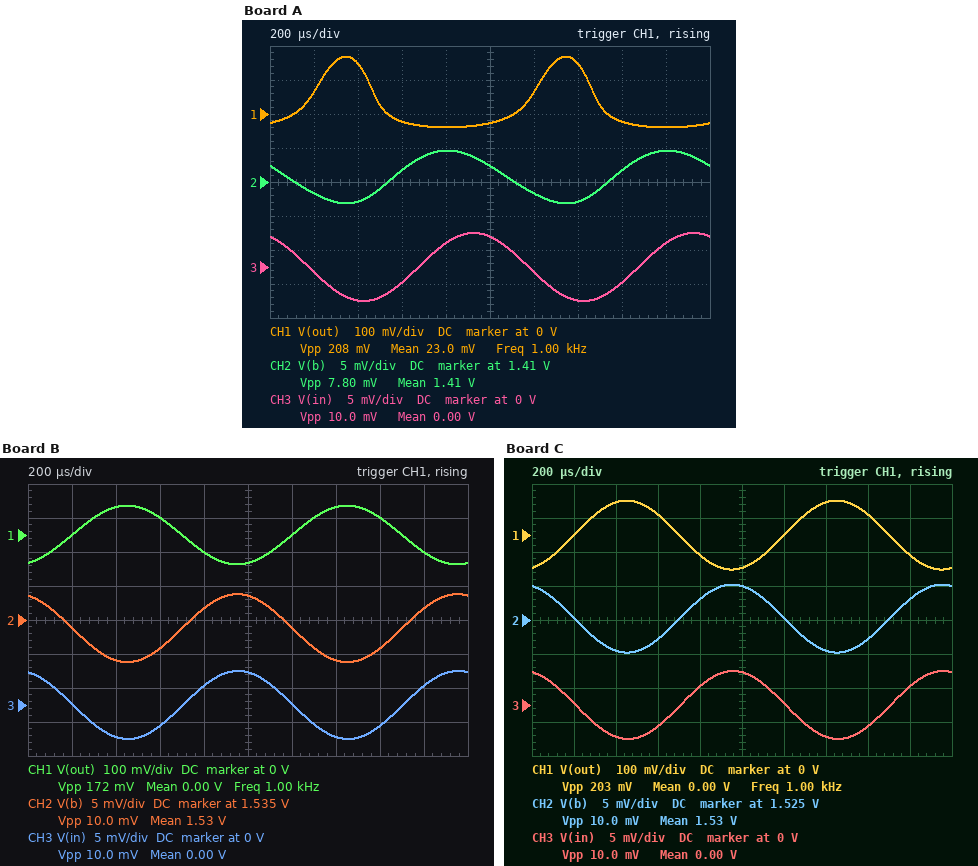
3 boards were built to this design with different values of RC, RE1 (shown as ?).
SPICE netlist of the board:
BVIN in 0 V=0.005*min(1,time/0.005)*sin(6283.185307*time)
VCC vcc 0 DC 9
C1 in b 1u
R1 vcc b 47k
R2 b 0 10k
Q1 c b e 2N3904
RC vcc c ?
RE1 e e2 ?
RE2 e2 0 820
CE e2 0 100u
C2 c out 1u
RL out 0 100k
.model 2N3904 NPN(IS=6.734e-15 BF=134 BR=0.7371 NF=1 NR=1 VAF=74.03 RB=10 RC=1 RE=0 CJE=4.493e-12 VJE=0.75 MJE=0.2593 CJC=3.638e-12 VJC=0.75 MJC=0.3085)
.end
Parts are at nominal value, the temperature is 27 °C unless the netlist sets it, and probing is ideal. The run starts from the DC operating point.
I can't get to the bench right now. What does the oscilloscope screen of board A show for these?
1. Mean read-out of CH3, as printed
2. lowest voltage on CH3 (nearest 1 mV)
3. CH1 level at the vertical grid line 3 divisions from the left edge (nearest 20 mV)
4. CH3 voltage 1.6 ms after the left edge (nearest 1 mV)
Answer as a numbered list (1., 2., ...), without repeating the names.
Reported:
1. 0.00 V
2. -5 mV
3. -20 mV
4. -2 mV
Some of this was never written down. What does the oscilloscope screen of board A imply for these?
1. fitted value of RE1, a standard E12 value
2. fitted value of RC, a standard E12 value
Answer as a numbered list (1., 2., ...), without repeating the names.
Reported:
1. 82 Ω
2. 10 kΩ
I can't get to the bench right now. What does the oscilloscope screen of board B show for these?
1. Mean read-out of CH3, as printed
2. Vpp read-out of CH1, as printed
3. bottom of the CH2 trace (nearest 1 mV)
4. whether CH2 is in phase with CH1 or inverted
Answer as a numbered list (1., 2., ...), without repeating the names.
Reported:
1. 0.00 V
2. 172 mV
3. 1.529 V
4. inverted
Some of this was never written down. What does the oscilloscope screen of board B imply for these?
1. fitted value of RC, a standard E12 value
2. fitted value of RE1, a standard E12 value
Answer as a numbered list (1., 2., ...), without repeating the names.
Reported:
1. 6.8 kΩ
2. 330 Ω
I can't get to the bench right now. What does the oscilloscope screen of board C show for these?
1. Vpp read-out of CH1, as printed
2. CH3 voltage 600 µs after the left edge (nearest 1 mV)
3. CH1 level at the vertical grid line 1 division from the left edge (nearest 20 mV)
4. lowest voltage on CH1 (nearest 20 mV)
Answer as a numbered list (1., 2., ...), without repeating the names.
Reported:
1. 203 mV
2. -3 mV
3. 0 V
4. -100 mV
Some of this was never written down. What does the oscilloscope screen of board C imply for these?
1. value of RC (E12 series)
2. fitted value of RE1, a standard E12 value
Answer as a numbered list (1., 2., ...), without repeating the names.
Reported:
1. 2.7 kΩ
2. 100 Ω
